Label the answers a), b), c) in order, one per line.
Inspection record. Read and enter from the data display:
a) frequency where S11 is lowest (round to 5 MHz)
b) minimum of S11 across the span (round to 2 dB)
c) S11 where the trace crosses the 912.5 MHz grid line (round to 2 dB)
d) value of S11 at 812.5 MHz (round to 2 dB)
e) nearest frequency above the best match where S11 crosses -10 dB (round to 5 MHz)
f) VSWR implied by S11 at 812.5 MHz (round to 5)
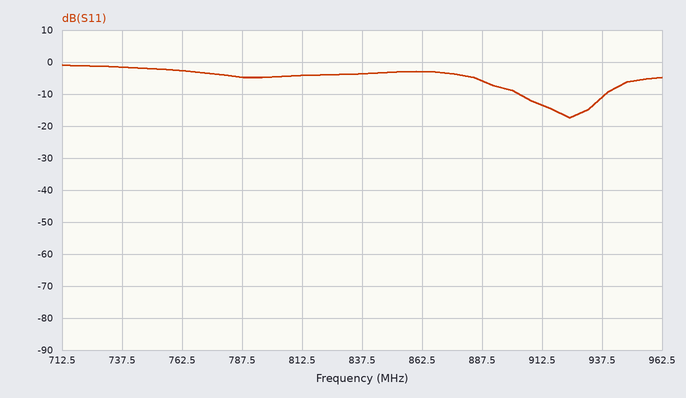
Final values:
a) 925 MHz
b) -18 dB
c) -14 dB
d) -4 dB
e) 940 MHz
f) 5
